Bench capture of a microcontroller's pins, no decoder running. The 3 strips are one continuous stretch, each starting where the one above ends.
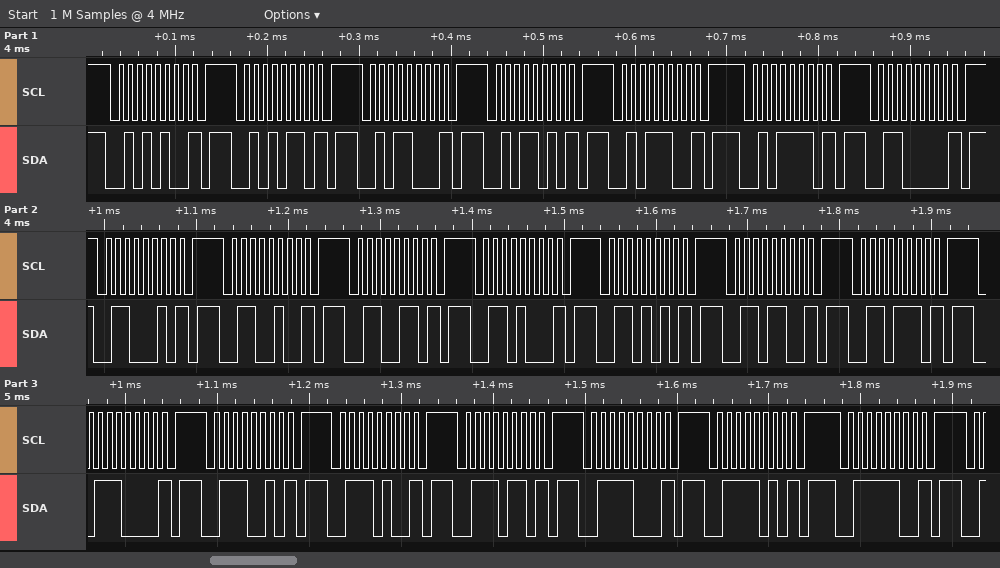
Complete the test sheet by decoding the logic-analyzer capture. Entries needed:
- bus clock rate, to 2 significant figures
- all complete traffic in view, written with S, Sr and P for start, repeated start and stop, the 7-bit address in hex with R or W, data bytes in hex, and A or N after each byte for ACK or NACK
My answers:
100 kHz
S 2AW N P S 2BW N P S 2CW N P S 2DW N P S 2EW N P S 2FW N P S 30W N P S 31W N P S 32W N P S 33W N P S 34W N P S 35W N P S 36W N P S 37W N P S 38W N P S 39W N P S 3AW N P S 3BW N P S 3CW N P S 3DW N P S 3EW N P
